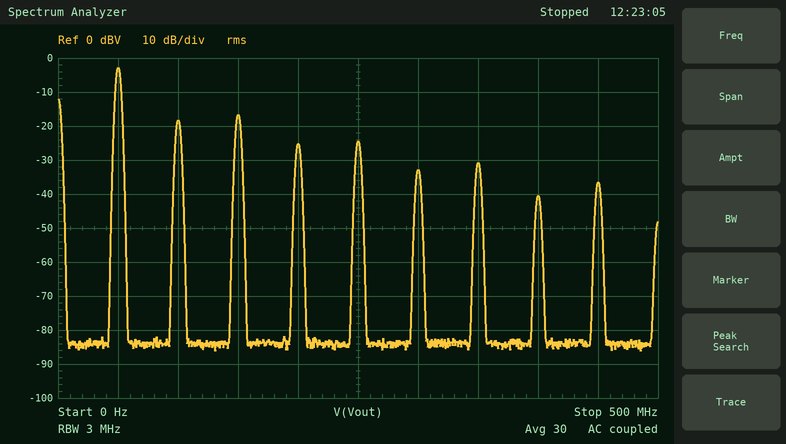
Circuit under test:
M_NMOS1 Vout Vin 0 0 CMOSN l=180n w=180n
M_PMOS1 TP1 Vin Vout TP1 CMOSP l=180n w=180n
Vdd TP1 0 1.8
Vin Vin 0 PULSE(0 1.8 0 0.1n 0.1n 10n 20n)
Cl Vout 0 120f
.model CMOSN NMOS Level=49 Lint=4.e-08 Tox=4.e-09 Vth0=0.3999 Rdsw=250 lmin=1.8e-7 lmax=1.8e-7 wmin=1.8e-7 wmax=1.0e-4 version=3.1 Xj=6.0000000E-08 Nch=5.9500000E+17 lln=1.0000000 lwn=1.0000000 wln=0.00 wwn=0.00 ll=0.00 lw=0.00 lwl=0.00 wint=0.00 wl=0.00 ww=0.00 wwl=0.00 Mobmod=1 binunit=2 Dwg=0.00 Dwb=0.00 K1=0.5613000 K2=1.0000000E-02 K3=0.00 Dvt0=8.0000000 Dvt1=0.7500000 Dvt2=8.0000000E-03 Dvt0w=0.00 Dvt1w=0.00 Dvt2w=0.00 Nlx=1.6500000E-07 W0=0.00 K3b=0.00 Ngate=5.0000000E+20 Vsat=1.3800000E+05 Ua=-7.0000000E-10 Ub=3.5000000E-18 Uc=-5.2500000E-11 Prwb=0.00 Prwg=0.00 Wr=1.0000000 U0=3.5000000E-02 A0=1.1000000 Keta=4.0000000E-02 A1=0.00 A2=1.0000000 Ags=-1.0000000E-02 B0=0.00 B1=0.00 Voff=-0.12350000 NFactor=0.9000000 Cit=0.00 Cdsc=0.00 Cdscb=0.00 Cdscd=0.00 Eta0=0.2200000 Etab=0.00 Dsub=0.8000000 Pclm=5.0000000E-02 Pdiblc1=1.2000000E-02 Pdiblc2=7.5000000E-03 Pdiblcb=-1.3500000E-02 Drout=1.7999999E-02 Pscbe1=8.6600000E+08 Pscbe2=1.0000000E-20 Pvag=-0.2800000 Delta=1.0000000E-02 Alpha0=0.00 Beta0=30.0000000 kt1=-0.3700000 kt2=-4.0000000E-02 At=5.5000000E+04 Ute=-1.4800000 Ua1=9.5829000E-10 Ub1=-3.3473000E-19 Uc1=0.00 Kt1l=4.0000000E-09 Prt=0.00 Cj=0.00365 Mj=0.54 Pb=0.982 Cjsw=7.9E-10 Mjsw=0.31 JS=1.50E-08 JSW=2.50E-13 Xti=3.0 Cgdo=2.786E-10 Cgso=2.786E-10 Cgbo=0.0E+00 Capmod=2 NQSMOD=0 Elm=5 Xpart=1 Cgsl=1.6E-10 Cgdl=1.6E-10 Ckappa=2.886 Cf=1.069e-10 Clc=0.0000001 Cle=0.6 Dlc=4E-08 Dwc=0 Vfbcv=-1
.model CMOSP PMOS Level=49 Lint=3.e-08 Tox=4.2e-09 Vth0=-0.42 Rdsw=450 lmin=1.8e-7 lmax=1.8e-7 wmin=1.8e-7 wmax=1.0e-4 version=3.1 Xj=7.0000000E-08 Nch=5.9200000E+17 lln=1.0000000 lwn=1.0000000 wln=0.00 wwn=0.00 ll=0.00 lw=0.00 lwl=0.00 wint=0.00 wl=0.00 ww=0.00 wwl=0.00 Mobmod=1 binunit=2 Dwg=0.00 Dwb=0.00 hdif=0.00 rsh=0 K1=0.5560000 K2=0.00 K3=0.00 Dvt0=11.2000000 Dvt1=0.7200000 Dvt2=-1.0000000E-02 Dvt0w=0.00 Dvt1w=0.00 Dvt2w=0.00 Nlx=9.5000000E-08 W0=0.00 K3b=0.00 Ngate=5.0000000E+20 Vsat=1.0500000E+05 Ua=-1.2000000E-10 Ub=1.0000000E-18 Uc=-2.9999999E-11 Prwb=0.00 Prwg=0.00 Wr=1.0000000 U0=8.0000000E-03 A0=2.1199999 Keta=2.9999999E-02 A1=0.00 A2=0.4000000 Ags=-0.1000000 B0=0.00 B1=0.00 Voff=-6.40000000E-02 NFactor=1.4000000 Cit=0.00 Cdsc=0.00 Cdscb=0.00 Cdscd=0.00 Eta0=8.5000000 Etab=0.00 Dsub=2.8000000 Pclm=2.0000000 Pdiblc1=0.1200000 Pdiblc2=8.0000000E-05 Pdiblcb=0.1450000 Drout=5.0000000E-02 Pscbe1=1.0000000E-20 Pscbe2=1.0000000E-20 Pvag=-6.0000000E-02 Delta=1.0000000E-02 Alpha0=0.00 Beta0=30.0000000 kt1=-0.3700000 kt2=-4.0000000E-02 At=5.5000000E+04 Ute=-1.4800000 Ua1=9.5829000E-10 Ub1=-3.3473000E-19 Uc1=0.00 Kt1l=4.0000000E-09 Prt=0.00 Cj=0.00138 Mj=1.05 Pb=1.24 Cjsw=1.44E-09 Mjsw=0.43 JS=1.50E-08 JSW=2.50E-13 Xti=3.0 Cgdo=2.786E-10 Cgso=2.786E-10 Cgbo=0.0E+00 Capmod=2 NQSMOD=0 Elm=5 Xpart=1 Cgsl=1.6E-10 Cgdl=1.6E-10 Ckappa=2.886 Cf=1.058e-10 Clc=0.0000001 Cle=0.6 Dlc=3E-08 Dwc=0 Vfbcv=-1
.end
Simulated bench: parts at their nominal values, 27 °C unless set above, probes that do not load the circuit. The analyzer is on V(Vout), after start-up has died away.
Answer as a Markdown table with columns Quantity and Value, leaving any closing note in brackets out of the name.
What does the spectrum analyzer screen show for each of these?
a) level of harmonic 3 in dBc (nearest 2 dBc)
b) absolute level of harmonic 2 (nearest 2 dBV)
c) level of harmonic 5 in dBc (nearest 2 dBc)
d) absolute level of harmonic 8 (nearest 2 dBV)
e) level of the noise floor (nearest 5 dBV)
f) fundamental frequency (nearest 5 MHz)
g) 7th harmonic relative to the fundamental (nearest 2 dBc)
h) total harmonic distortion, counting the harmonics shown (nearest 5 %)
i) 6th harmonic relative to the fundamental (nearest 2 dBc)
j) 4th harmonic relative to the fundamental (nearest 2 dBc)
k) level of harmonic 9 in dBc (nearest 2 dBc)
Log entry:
| Quantity | Value |
|---|---|
| level of harmonic 3 in dBc | -14 dBc |
| absolute level of harmonic 2 | -18 dBV |
| level of harmonic 5 in dBc | -22 dBc |
| absolute level of harmonic 8 | -40 dBV |
| level of the noise floor | -85 dBV |
| fundamental frequency | 50 MHz |
| 7th harmonic relative to the fundamental | -28 dBc |
| total harmonic distortion, counting the harmonics shown | 30 % |
| 6th harmonic relative to the fundamental | -30 dBc |
| 4th harmonic relative to the fundamental | -22 dBc |
| level of harmonic 9 in dBc | -34 dBc |
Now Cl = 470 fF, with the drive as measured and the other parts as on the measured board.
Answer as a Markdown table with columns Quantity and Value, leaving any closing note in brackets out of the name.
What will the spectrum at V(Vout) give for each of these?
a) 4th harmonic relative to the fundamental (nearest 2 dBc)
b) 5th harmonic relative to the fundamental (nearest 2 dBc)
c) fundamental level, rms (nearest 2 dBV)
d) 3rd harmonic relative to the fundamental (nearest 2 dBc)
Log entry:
| Quantity | Value |
|---|---|
| 4th harmonic relative to the fundamental | -30 dBc |
| 5th harmonic relative to the fundamental | -28 dBc |
| fundamental level, rms | -10 dBV |
| 3rd harmonic relative to the fundamental | -18 dBc |
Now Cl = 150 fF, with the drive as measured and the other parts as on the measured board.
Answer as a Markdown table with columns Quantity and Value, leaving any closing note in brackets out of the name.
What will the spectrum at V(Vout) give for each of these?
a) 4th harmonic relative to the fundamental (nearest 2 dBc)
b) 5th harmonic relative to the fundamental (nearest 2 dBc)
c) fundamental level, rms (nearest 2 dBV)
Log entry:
| Quantity | Value |
|---|---|
| 4th harmonic relative to the fundamental | -24 dBc |
| 5th harmonic relative to the fundamental | -24 dBc |
| fundamental level, rms | -4 dBV |
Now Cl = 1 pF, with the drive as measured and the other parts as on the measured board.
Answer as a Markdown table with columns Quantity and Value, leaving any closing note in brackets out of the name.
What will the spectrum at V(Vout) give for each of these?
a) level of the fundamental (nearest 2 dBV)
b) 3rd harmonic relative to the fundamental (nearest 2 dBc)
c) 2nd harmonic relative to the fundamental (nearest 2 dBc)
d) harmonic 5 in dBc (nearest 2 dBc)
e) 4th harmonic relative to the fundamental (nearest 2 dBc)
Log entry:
| Quantity | Value |
|---|---|
| level of the fundamental | -16 dBV |
| 3rd harmonic relative to the fundamental | -18 dBc |
| 2nd harmonic relative to the fundamental | -20 dBc |
| harmonic 5 in dBc | -28 dBc |
| 4th harmonic relative to the fundamental | -32 dBc |
